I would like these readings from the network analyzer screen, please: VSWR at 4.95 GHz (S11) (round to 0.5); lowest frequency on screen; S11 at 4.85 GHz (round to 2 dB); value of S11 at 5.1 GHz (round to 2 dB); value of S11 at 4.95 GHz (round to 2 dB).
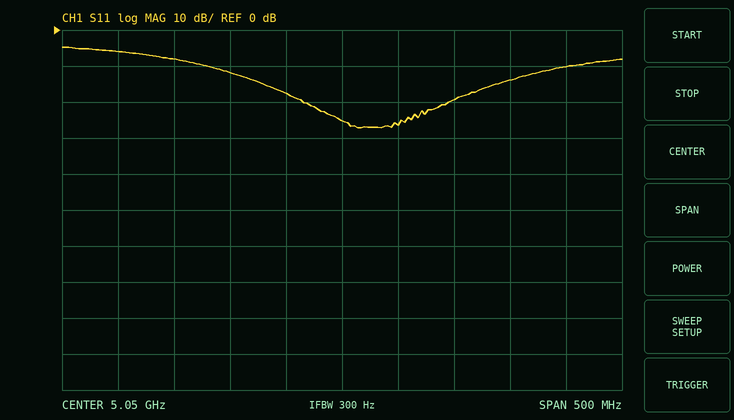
1.5
4.8 GHz
-6 dB
-26 dB
-12 dB
